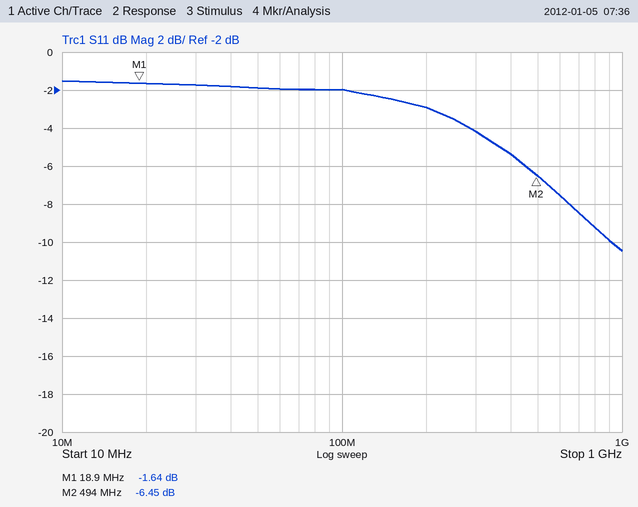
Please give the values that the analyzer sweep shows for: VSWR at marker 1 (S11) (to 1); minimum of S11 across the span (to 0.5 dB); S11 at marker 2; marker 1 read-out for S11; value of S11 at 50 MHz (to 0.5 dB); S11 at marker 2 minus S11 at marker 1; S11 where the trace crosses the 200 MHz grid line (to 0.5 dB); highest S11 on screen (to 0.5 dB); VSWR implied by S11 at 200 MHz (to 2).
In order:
11
-10.5 dB
-6.45 dB
-1.64 dB
-2.0 dB
-4.81 dB
-3.0 dB
-1.5 dB
6
